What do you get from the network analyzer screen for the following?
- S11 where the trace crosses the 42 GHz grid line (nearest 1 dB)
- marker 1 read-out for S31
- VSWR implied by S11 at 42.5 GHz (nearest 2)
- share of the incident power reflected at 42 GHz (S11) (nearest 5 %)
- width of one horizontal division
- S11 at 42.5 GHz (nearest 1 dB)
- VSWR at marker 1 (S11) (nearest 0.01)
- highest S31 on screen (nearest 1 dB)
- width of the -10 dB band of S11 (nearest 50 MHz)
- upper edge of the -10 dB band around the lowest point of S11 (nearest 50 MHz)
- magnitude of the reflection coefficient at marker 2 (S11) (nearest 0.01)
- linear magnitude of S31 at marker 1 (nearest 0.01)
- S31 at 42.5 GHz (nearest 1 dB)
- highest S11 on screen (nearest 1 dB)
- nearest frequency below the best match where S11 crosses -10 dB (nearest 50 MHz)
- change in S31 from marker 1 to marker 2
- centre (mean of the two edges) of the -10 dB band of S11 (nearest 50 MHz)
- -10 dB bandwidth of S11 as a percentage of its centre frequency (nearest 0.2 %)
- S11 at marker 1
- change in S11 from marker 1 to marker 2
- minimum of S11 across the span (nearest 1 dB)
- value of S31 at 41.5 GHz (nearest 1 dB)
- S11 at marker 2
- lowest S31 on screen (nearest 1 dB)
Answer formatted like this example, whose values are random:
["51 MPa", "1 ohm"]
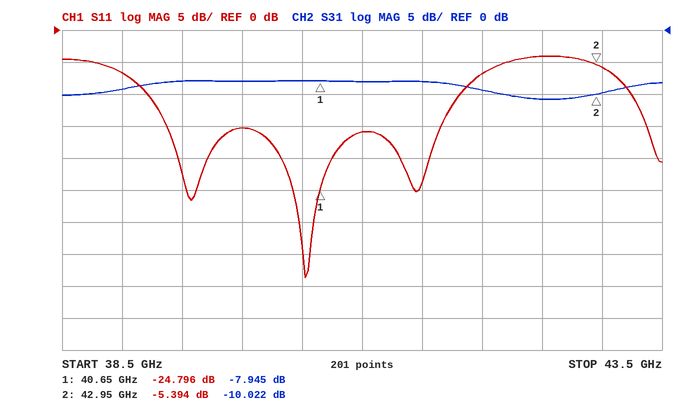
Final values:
["-7 dB", "-7.945 dB", "4", "20 %", "500 MHz", "-4 dB", "1.12", "-8 dB", "2.60 GHz", "41.80 GHz", "0.54", "0.40", "-11 dB", "-4 dB", "39.20 GHz", "-2.077 dB", "40.50 GHz", "6.4 %", "-24.796 dB", "19.402 dB", "-39 dB", "-8 dB", "-5.394 dB", "-11 dB"]
